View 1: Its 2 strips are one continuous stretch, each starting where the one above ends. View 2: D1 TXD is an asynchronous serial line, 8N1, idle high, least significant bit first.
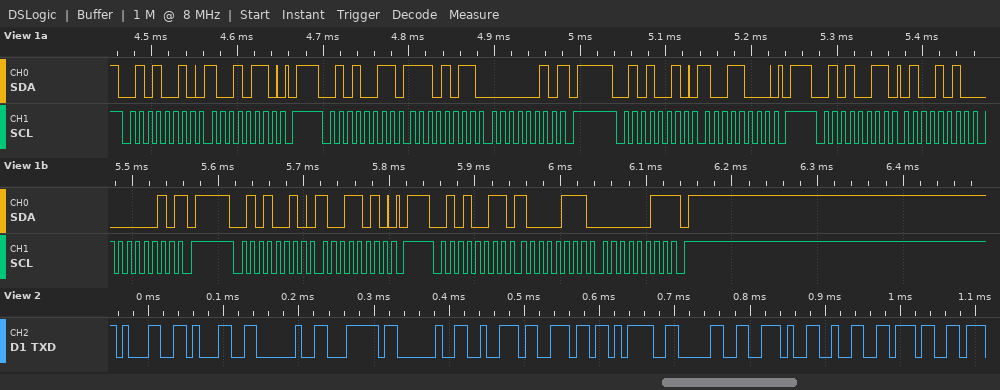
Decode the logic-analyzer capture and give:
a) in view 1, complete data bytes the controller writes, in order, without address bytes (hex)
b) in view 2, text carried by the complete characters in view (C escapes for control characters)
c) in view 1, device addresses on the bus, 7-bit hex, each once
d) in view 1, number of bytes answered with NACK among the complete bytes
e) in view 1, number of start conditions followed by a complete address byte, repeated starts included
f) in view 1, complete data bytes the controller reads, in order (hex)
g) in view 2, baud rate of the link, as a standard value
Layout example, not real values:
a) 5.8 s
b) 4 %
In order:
a) 96 98 9A
b) "11 | rn=0.27"
c) 0x29
d) 3
e) 6
f) EB 02 4A 02 87 03
g) 115200 baud
